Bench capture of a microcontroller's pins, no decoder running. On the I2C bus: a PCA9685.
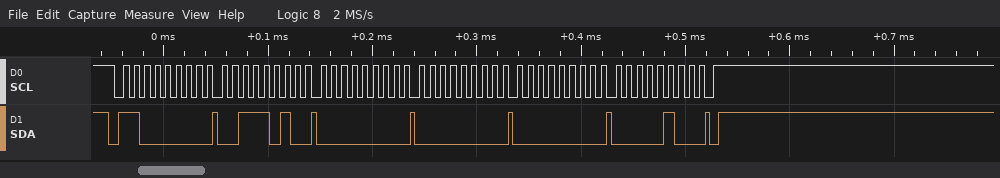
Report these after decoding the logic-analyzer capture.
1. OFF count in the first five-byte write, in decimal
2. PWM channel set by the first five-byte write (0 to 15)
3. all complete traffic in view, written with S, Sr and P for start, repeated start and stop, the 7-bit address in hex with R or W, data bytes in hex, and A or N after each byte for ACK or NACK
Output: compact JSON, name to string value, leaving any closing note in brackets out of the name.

{"OFF count in the first five-byte write, in decimal": "1024", "PWM channel set by the first five-byte write": "13", "all complete traffic in view, written with S, Sr and P for start, repeated start and stop, the 7-bit address in hex with R or W, data bytes in hex, and A or N after each byte for ACK or NACK": "S 60W A 3A A 00 A 00 A 00 A 04 A P"}
